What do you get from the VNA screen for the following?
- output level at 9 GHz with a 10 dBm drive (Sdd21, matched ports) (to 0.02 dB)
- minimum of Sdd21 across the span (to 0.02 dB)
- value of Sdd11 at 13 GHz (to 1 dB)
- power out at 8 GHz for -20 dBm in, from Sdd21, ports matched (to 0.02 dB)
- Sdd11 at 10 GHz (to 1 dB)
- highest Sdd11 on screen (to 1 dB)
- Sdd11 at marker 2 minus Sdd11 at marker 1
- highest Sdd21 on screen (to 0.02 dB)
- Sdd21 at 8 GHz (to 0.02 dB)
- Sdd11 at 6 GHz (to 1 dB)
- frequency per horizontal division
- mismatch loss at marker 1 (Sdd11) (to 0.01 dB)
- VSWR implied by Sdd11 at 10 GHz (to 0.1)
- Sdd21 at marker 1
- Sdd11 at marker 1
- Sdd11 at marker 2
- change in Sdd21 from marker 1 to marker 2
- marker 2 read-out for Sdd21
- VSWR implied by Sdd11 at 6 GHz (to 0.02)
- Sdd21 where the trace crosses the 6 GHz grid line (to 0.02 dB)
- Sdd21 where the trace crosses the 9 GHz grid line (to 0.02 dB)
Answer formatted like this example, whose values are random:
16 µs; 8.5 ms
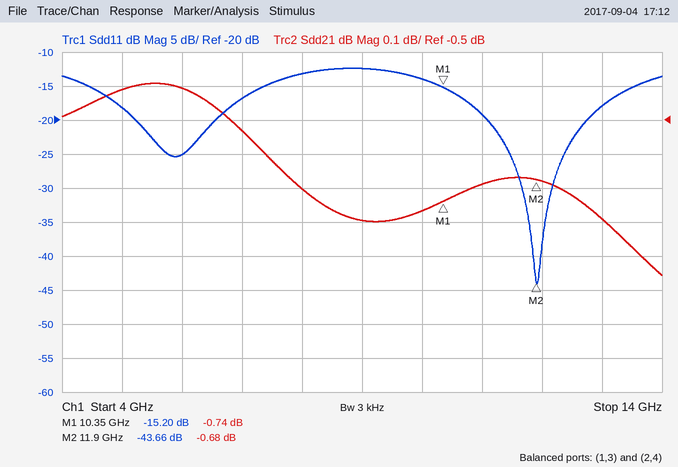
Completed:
9.20 dBm; -0.96 dB; -18 dB; -20.70 dBm; -14 dB; -12 dB; -28.46 dB; -0.40 dB; -0.70 dB; -25 dB; 1 GHz; 0.13 dB; 1.5; -0.74 dB; -15.20 dB; -43.66 dB; 0.06 dB; -0.68 dB; 1.12; -0.40 dB; -0.80 dB
